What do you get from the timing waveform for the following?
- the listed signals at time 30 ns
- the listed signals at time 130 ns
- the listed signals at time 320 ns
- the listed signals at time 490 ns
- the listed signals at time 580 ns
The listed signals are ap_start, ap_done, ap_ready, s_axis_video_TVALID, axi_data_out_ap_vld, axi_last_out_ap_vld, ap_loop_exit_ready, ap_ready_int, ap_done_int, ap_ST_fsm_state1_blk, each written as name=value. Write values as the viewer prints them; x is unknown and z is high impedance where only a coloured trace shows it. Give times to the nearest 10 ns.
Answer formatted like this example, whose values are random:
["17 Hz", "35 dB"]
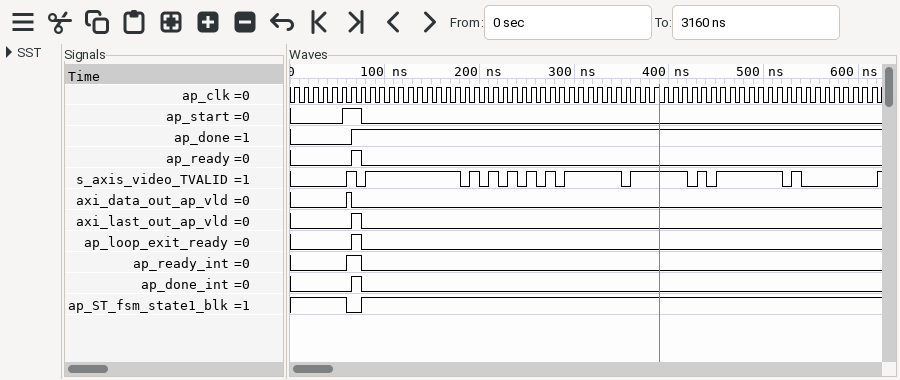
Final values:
["ap_start=0, ap_done=0, ap_ready=0, s_axis_video_TVALID=0, axi_data_out_ap_vld=0, axi_last_out_ap_vld=0, ap_loop_exit_ready=0, ap_ready_int=0, ap_done_int=0, ap_ST_fsm_state1_blk=1", "ap_start=0, ap_done=1, ap_ready=0, s_axis_video_TVALID=1, axi_data_out_ap_vld=0, axi_last_out_ap_vld=0, ap_loop_exit_ready=0, ap_ready_int=0, ap_done_int=0, ap_ST_fsm_state1_blk=1", "ap_start=0, ap_done=1, ap_ready=0, s_axis_video_TVALID=1, axi_data_out_ap_vld=0, axi_last_out_ap_vld=0, ap_loop_exit_ready=0, ap_ready_int=0, ap_done_int=0, ap_ST_fsm_state1_blk=1", "ap_start=0, ap_done=1, ap_ready=0, s_axis_video_TVALID=1, axi_data_out_ap_vld=0, axi_last_out_ap_vld=0, ap_loop_exit_ready=0, ap_ready_int=0, ap_done_int=0, ap_ST_fsm_state1_blk=1", "ap_start=0, ap_done=1, ap_ready=0, s_axis_video_TVALID=0, axi_data_out_ap_vld=0, axi_last_out_ap_vld=0, ap_loop_exit_ready=0, ap_ready_int=0, ap_done_int=0, ap_ST_fsm_state1_blk=1"]
